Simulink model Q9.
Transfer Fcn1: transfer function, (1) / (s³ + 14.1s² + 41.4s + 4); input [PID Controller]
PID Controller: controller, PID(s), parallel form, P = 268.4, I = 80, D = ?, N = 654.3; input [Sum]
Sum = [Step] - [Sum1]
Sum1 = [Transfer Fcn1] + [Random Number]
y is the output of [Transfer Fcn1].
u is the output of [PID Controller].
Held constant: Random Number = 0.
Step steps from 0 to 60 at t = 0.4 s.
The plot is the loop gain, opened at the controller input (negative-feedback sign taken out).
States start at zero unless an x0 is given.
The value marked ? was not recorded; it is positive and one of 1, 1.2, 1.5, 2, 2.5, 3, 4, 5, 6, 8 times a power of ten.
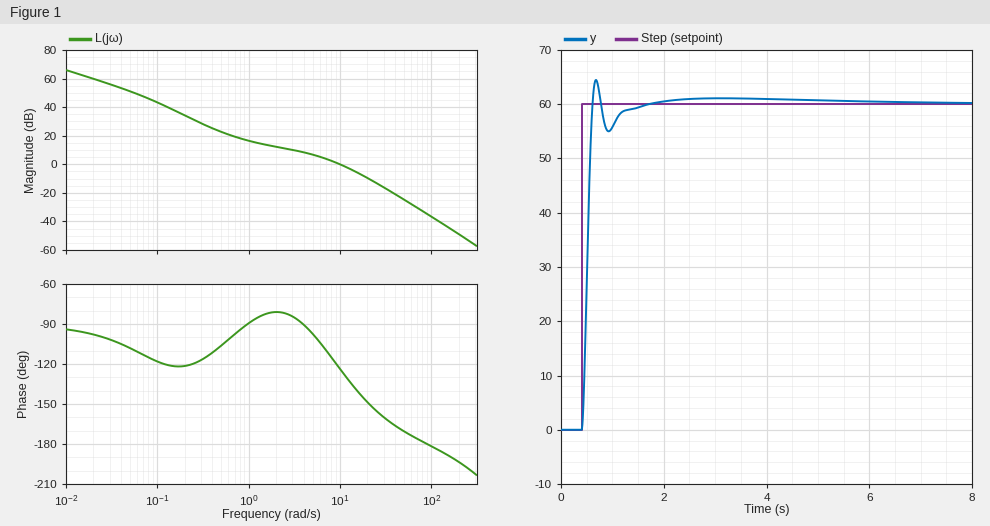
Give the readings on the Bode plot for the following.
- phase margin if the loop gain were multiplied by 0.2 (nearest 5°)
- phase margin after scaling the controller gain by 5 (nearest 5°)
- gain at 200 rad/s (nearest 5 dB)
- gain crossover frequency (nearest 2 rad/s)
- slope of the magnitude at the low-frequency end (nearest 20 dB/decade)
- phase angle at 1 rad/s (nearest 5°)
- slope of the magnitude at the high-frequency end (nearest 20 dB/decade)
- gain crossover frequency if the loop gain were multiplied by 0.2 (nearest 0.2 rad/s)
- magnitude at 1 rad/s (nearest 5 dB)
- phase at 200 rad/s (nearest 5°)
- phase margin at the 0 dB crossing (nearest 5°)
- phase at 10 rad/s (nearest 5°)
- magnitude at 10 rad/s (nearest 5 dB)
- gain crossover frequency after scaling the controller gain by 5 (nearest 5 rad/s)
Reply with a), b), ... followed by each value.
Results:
a) 95°
b) 25°
c) -50 dB
d) 10 rad/s
e) -20 dB/decade
f) -90°
g) -40 dB/decade
h) 1.4 rad/s
i) 15 dB
j) -195°
k) 55°
l) -125°
m) 0 dB
n) 25 rad/s
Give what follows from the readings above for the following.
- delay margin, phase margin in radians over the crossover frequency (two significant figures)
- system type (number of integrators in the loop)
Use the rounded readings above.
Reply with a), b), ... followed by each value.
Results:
a) 0.096 s
b) 1
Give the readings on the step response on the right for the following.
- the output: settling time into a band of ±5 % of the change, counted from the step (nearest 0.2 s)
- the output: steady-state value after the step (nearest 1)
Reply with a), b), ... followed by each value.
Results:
a) 0.6 s
b) 60
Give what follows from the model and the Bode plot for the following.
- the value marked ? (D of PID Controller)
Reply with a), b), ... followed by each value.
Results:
a) 150
